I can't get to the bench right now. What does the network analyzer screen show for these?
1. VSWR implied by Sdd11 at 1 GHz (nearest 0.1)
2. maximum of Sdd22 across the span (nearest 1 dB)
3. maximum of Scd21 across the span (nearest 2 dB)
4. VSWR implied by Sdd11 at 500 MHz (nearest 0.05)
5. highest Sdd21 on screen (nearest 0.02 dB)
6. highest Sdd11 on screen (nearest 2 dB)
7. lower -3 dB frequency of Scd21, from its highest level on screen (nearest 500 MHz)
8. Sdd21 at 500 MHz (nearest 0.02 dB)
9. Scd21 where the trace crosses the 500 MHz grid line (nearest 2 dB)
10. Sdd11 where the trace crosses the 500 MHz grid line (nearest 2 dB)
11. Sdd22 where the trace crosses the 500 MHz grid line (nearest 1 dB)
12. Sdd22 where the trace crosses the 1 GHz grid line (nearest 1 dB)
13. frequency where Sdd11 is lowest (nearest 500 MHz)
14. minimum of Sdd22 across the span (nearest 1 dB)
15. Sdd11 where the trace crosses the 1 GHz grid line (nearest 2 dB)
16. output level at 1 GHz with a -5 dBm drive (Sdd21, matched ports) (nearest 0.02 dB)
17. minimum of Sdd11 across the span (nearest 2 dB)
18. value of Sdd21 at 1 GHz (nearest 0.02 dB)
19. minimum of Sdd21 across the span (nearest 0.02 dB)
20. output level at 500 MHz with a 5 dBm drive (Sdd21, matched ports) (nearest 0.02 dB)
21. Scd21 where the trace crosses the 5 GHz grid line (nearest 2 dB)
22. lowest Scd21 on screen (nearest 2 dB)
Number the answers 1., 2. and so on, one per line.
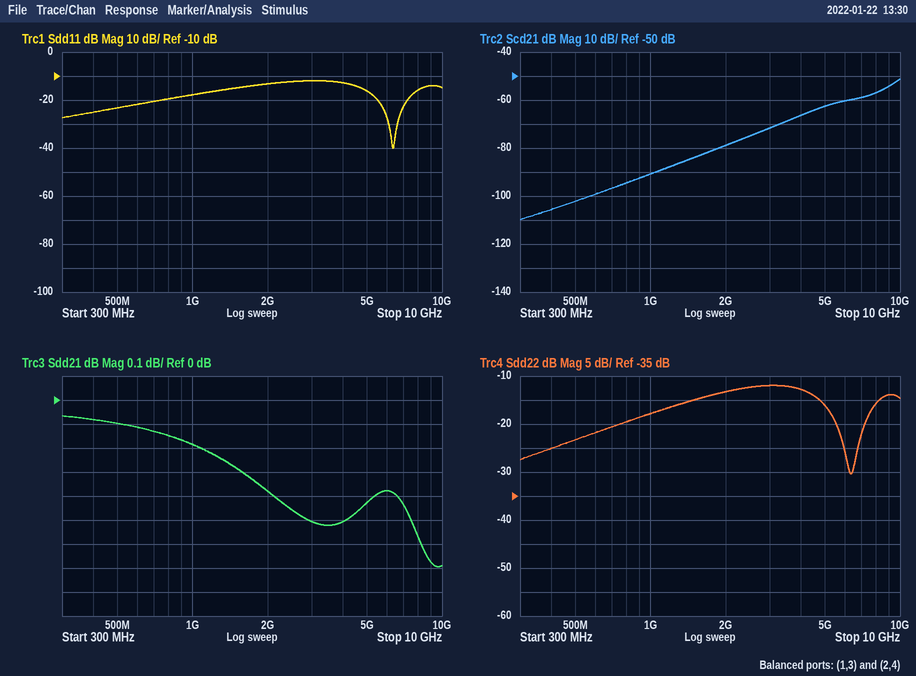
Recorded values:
1. 1.3
2. -12 dB
3. -52 dB
4. 1.15
5. -0.06 dB
6. -12 dB
7. 9.0 GHz
8. -0.10 dB
9. -102 dB
10. -24 dB
11. -23 dB
12. -18 dB
13. 6.5 GHz
14. -30 dB
15. -18 dB
16. -5.18 dBm
17. -40 dB
18. -0.18 dB
19. -0.70 dB
20. 4.90 dBm
21. -62 dB
22. -110 dB
